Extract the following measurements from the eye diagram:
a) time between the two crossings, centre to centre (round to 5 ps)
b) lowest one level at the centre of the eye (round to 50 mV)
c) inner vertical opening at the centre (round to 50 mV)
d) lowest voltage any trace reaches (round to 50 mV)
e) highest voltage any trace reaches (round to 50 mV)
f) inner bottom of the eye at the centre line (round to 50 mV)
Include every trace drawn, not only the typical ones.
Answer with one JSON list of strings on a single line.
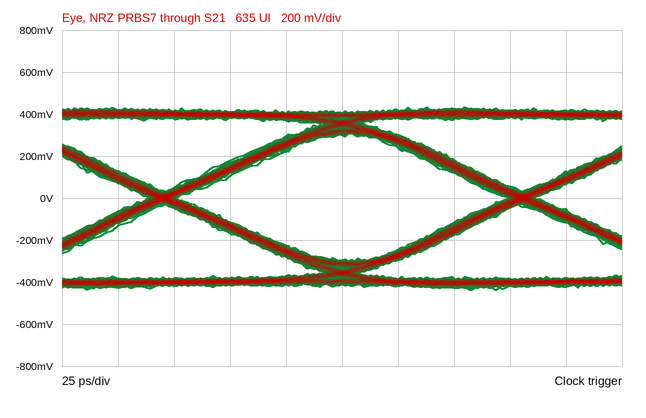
["160 ps", "300 mV", "600 mV", "-450 mV", "450 mV", "-300 mV"]
